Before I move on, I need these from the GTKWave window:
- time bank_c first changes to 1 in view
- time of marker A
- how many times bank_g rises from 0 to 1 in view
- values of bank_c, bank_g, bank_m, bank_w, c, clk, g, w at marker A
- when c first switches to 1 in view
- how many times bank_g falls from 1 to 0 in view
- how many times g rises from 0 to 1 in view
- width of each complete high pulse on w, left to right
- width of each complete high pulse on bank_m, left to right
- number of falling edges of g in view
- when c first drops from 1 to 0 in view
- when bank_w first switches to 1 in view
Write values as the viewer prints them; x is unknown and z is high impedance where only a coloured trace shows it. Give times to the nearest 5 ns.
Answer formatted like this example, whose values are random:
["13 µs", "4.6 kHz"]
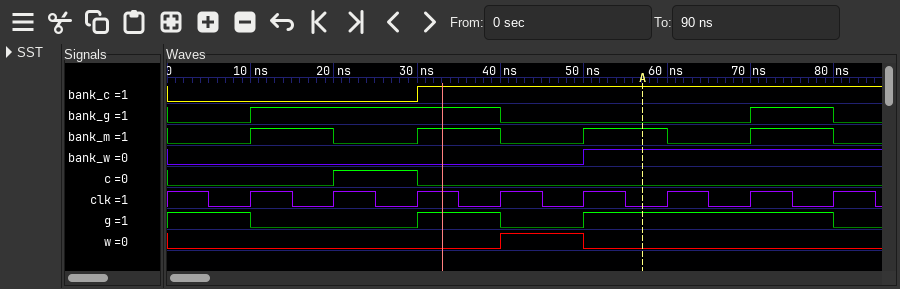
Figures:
["30 ns", "55 ns", "2", "bank_c=1, bank_g=0, bank_m=1, bank_w=1, c=0, clk=0, g=1, w=0", "20 ns", "2", "2", "10 ns", "10 ns, 10 ns, 10 ns, 10 ns", "3", "30 ns", "50 ns"]
